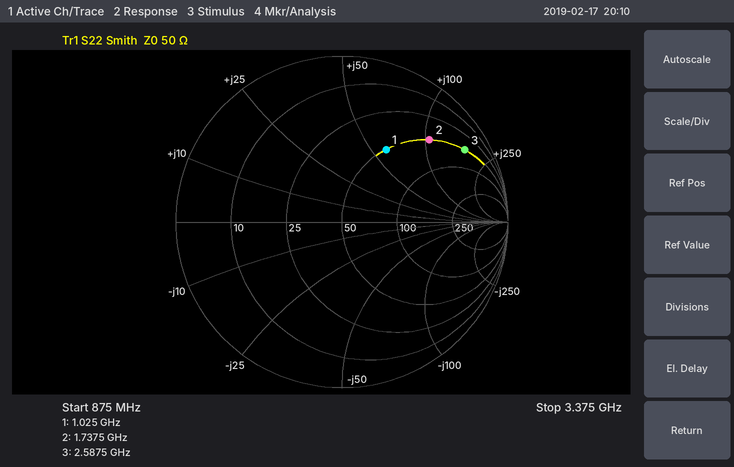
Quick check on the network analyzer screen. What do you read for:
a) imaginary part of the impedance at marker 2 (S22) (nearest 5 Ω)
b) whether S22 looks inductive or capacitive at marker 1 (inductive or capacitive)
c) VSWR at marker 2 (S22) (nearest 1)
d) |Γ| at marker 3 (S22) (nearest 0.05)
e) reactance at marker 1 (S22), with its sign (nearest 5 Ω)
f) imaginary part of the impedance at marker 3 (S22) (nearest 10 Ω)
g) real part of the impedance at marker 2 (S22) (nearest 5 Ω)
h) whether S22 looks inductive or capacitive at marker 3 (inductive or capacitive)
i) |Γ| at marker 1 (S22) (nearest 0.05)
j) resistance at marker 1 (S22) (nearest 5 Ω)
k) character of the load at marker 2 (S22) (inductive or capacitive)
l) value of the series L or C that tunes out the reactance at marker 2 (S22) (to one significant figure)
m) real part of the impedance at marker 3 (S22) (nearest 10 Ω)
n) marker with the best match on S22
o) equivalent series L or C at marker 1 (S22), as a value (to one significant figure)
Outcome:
+105 Ω
inductive
6
0.85
+60 Ω
+170 Ω
50 Ω
inductive
0.50
50 Ω
inductive
900 fF
50 Ω
marker 1
9 nH
